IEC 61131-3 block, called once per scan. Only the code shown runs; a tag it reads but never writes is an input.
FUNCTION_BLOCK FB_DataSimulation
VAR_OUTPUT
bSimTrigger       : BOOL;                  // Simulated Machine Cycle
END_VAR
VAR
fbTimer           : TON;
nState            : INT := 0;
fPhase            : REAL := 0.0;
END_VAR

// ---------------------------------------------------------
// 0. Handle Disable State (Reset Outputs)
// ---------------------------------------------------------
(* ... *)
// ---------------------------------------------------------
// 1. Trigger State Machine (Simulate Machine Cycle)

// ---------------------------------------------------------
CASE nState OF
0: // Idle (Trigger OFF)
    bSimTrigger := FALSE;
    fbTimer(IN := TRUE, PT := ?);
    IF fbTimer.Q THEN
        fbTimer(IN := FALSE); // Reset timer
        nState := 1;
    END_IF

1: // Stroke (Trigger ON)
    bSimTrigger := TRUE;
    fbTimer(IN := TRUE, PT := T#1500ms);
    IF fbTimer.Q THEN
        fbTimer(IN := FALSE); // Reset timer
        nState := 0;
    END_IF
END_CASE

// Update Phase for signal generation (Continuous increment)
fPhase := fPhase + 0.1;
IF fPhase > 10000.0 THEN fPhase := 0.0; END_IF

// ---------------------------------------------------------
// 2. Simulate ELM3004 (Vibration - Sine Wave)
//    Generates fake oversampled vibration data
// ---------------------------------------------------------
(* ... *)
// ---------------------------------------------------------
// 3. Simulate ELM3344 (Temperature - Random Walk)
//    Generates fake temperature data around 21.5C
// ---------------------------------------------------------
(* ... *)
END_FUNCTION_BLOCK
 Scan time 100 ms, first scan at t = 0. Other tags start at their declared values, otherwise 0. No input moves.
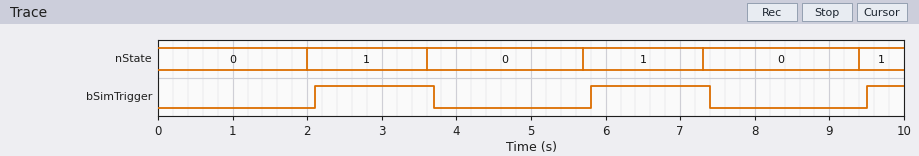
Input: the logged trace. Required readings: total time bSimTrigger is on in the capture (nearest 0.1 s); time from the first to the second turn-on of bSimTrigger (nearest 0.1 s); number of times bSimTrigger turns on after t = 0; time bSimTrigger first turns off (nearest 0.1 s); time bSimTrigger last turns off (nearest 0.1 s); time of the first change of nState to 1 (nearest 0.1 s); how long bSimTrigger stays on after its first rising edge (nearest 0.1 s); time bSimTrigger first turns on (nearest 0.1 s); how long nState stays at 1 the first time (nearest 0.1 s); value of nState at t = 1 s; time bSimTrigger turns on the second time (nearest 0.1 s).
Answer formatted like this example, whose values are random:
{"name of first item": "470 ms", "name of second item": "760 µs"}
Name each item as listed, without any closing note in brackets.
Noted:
{"total time bSimTrigger is on in the capture": "3.7 s", "time from the first to the second turn-on of bSimTrigger": "3.7 s", "number of times bSimTrigger turns on after t = 0": "3", "time bSimTrigger first turns off": "3.7 s", "time bSimTrigger last turns off": "7.4 s", "time of the first change of nState to 1": "2.0 s", "how long bSimTrigger stays on after its first rising edge": "1.6 s", "time bSimTrigger first turns on": "2.1 s", "how long nState stays at 1 the first time": "1.6 s", "value of nState at t = 1 s": "0", "time bSimTrigger turns on the second time": "5.8 s"}
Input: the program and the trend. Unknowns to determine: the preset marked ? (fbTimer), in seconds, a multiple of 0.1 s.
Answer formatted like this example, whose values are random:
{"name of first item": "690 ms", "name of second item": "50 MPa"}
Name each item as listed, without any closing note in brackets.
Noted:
{"the preset marked ? (fbTimer), in seconds, a multiple of 0.1 s": "2.0 s"}
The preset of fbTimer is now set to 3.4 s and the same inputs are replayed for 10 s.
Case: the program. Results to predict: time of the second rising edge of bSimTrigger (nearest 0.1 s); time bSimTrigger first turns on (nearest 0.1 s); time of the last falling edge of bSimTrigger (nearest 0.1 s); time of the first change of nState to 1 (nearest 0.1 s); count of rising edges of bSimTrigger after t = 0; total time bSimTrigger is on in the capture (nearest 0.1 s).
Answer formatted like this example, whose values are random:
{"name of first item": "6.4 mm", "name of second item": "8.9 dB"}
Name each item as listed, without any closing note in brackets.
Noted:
{"time of the second rising edge of bSimTrigger": "8.6 s", "time bSimTrigger first turns on": "3.5 s", "time of the last falling edge of bSimTrigger": "5.1 s", "time of the first change of nState to 1": "3.4 s", "count of rising edges of bSimTrigger after t = 0": "2", "total time bSimTrigger is on in the capture": "3.0 s"}
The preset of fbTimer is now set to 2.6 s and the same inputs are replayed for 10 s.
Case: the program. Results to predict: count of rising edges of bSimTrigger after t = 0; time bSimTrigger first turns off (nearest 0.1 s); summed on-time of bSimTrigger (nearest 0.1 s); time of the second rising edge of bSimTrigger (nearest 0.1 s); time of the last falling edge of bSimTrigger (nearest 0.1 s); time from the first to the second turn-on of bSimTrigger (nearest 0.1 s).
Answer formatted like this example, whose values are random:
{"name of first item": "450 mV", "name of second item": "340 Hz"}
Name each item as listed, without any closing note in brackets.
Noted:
{"count of rising edges of bSimTrigger after t = 0": "2", "time bSimTrigger first turns off": "4.3 s", "summed on-time of bSimTrigger": "3.2 s", "time of the second rising edge of bSimTrigger": "7.0 s", "time of the last falling edge of bSimTrigger": "8.6 s", "time from the first to the second turn-on of bSimTrigger": "4.3 s"}
